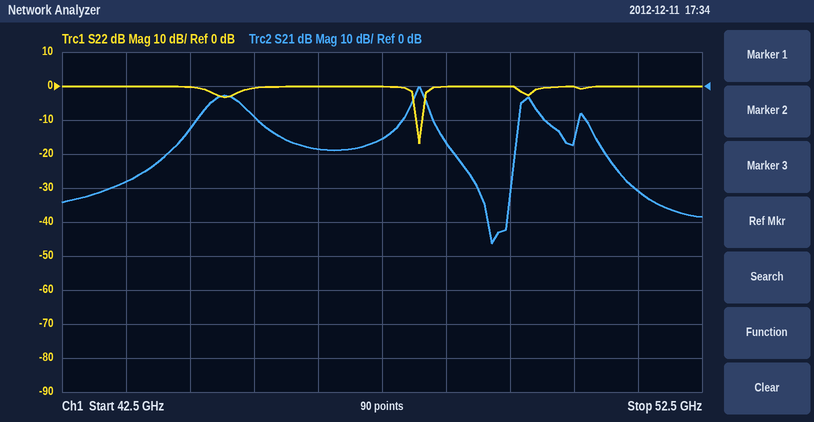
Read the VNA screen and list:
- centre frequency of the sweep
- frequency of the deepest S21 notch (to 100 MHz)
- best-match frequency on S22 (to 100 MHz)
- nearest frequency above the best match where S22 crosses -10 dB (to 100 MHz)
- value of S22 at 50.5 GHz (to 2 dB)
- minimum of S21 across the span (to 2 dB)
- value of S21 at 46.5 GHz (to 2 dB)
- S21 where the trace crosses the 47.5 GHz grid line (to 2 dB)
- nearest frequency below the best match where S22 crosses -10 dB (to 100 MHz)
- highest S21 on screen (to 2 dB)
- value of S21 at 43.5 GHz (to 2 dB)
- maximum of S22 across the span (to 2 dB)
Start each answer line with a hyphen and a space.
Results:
- 47.5 GHz
- 49.2 GHz
- 48.1 GHz
- 48.1 GHz
- 0 dB
- -46 dB
- -18 dB
- -16 dB
- 48.0 GHz
- 0 dB
- -28 dB
- 0 dB
